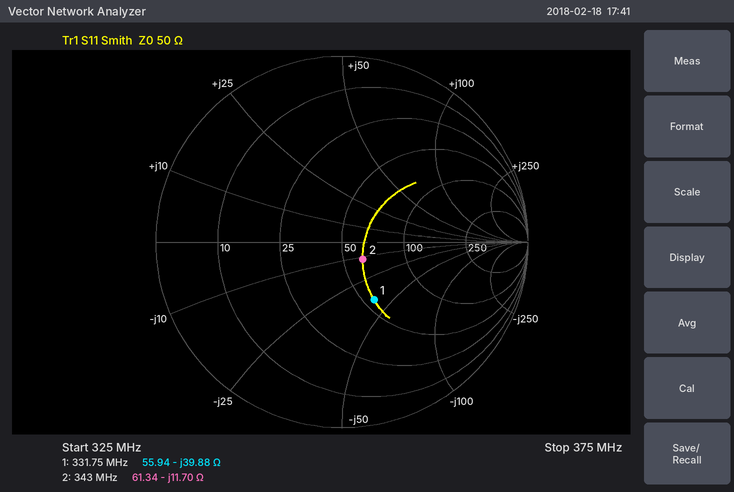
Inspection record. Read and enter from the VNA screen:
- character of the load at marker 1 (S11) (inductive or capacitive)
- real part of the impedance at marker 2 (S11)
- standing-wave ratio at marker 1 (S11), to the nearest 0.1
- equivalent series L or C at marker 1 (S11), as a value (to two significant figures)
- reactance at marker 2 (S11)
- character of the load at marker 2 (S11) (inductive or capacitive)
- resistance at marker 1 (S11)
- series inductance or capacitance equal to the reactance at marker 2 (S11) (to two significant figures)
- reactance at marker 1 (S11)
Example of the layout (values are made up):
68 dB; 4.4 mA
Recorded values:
capacitive; 61.34 Ω; 2.1; 12 pF; -11.70 Ω; capacitive; 55.94 Ω; 40 pF; -39.88 Ω
